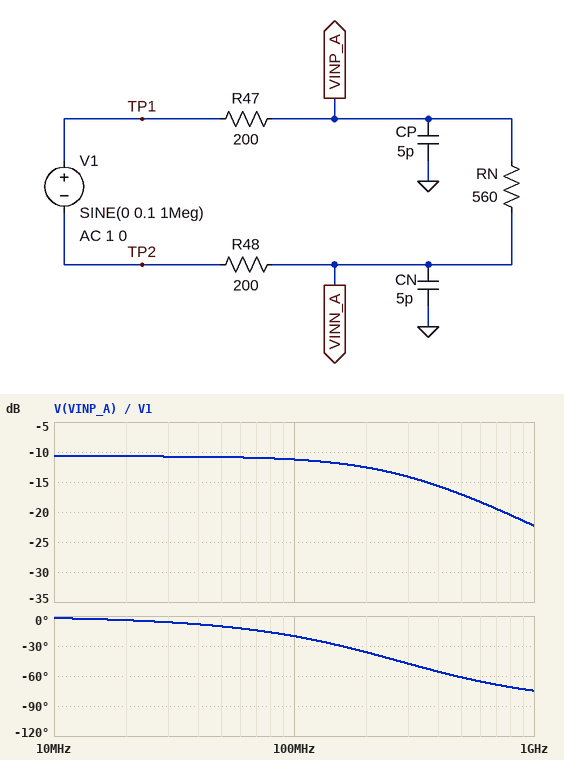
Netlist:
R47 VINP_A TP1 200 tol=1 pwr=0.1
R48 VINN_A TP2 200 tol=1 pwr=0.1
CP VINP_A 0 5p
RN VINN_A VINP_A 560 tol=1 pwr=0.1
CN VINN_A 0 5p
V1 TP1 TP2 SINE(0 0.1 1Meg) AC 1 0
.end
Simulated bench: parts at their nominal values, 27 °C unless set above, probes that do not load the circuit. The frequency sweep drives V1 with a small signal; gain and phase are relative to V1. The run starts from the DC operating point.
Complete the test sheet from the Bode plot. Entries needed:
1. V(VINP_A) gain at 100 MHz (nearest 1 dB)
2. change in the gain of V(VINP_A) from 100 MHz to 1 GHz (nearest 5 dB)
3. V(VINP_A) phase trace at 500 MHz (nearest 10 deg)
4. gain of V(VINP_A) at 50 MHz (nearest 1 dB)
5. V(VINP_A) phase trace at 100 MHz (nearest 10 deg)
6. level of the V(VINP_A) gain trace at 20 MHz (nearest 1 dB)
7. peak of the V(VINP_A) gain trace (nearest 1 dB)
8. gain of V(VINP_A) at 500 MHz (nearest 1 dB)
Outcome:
-11 dB
-10 dB
-60 deg
-11 dB
-20 deg
-11 dB
-11 dB
-17 dB
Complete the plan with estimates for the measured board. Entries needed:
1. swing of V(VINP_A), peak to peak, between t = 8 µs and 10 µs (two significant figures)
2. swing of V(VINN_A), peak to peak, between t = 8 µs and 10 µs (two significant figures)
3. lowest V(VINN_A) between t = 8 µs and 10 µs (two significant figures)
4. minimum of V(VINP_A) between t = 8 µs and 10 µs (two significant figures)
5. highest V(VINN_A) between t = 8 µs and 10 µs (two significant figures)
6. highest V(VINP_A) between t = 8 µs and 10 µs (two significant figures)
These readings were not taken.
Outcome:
58 mV
58 mV
-29 mV
-29 mV
29 mV
29 mV
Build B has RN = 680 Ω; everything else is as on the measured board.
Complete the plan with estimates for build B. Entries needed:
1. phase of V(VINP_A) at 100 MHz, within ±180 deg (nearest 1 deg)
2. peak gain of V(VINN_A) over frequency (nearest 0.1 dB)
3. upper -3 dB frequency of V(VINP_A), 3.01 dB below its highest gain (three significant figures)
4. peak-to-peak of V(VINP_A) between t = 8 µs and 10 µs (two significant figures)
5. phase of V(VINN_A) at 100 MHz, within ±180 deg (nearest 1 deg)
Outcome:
-22 deg
-10.0 dB
253 MHz
63 mV
158 deg
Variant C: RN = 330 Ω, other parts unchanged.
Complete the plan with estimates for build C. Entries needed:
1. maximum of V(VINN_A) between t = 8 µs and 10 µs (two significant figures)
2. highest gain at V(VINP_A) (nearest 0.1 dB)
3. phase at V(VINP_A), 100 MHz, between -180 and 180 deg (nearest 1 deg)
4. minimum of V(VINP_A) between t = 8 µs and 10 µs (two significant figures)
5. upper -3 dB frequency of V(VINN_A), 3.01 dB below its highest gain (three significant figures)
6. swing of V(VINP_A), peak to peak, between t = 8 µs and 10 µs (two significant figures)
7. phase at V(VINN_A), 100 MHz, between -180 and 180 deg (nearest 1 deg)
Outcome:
23 mV
-12.9 dB
-16 deg
-23 mV
352 MHz
45 mV
164 deg
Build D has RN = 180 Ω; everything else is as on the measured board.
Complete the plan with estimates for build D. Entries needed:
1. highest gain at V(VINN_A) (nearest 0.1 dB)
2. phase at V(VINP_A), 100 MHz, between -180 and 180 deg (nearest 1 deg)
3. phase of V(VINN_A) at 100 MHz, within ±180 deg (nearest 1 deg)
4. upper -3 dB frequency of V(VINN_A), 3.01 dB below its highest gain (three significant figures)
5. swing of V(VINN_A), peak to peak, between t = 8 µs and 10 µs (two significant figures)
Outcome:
-16.2 dB
-11 deg
169 deg
513 MHz
31 mV
